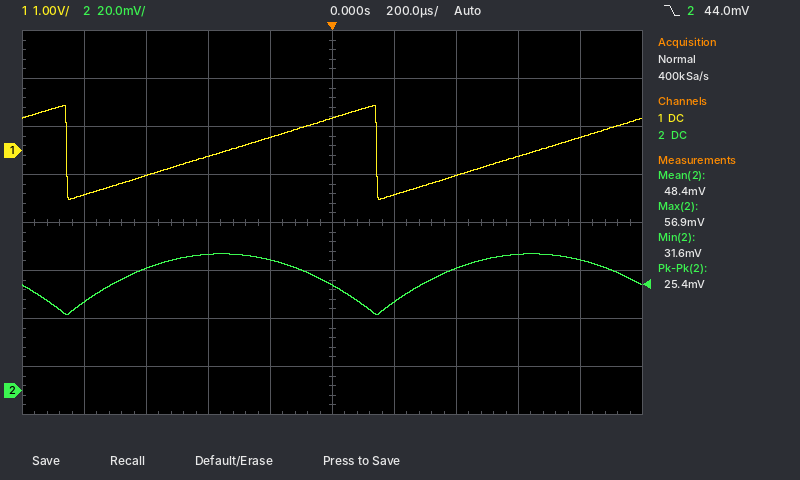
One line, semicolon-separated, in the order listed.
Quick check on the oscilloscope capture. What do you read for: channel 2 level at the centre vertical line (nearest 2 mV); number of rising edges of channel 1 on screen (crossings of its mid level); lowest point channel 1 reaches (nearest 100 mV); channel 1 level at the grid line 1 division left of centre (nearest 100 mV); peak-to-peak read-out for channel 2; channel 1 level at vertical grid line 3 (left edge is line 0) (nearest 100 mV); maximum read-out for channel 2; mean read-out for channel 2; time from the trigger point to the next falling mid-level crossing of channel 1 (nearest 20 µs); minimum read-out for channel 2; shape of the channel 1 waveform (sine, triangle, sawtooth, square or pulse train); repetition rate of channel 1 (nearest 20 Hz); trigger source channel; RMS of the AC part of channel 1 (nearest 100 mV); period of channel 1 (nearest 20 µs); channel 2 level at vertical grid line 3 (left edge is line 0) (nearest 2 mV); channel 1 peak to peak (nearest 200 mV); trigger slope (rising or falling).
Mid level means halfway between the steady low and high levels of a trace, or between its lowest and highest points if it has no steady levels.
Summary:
44 mV; 2; -1.0 V; 300 mV; 25.4 mV; -100 mV; 56.9 mV; 48.4 mV; 140 µs; 31.6 mV; sawtooth; 1.00 kHz; channel 2; 600 mV; 1.00 ms; 56 mV; 2.0 V; falling
